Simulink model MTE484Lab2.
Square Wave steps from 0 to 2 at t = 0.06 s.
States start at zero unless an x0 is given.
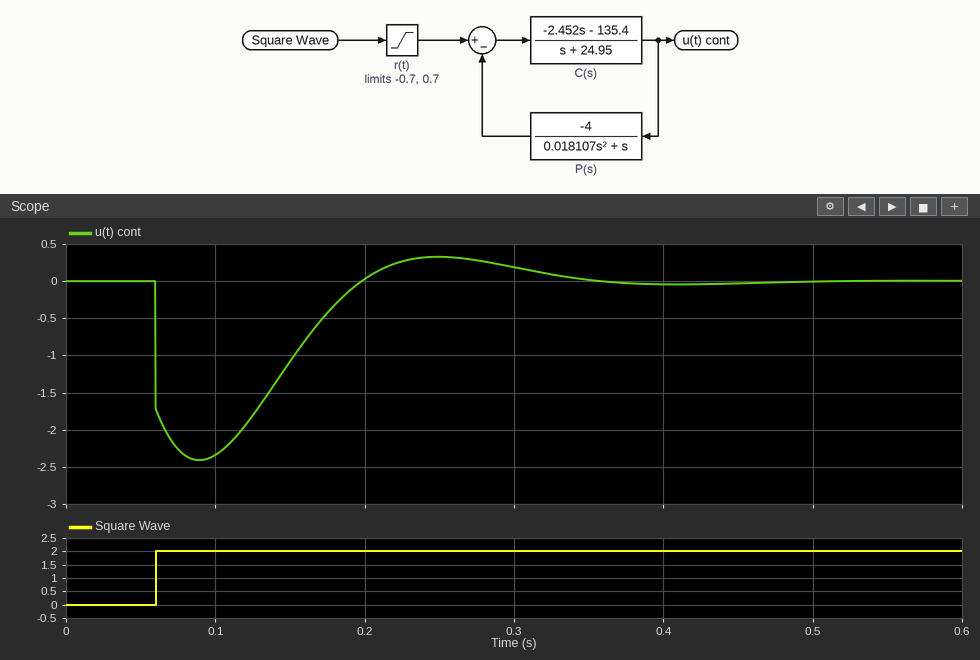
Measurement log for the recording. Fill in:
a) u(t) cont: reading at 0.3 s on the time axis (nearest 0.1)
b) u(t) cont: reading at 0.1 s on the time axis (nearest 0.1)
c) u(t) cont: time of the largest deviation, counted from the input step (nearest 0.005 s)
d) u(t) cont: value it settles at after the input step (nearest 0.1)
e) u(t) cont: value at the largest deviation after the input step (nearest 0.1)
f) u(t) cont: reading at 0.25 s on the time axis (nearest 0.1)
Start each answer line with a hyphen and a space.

- 0.2
- -2.3
- 0.030 s
- 0.0
- -2.4
- 0.3
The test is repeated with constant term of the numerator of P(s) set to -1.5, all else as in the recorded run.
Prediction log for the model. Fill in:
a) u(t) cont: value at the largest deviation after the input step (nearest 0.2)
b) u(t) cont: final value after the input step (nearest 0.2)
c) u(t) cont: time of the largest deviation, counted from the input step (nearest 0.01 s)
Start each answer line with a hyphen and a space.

- -2.8
- 0.0
- 0.05 s
